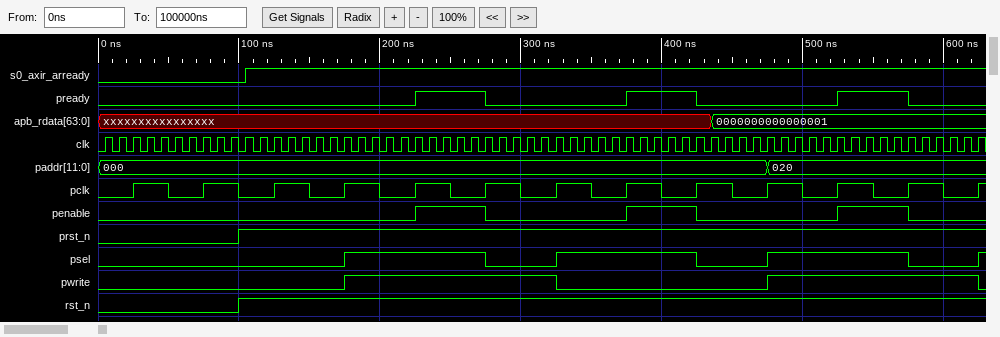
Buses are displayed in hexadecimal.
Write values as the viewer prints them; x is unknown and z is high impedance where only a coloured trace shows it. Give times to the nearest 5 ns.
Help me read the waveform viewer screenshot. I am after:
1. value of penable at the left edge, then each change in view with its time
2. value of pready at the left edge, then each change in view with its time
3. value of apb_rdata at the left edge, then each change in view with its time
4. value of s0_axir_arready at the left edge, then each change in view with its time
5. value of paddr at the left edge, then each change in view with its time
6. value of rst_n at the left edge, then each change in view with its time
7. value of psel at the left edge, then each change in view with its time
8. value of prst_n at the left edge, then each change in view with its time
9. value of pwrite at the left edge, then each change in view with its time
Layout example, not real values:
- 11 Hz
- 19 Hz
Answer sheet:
- 0, 1 at 225 ns, 0 at 275 ns, 1 at 375 ns, 0 at 425 ns, 1 at 525 ns, 0 at 575 ns
- 0, 1 at 225 ns, 0 at 275 ns, 1 at 375 ns, 0 at 425 ns, 1 at 525 ns, 0 at 575 ns
- xxxxxxxxxxxxxxxx, 0000000000000001 at 435 ns
- 0, 1 at 105 ns
- 000, 020 at 475 ns
- 0, 1 at 100 ns
- 0, 1 at 175 ns, 0 at 275 ns, 1 at 325 ns, 0 at 425 ns, 1 at 475 ns, 0 at 575 ns, 1 at 625 ns
- 0, 1 at 100 ns
- 0, 1 at 175 ns, 0 at 325 ns, 1 at 475 ns, 0 at 625 ns
